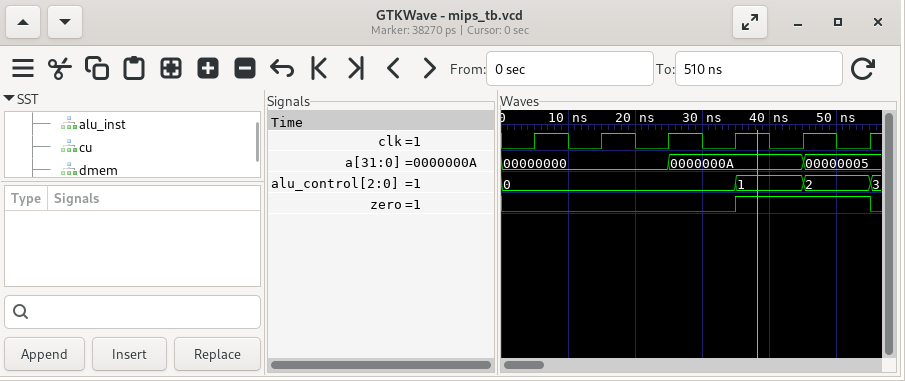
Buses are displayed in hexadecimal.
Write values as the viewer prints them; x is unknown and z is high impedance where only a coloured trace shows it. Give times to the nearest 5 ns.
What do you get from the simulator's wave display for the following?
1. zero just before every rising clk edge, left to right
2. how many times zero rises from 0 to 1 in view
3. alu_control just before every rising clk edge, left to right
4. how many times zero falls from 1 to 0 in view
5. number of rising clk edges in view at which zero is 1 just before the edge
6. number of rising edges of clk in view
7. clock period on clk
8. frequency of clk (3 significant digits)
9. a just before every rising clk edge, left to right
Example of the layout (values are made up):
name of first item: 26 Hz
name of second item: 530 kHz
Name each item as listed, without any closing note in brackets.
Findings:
zero just before every rising clk edge, left to right: 0 0 0 0 1 1
how many times zero rises from 0 to 1 in view: 1
alu_control just before every rising clk edge, left to right: 0, 0, 0, 0, 1, 2
how many times zero falls from 1 to 0 in view: 1
number of rising clk edges in view at which zero is 1 just before the edge: 2
number of rising edges of clk in view: 6
clock period on clk: 10 ns
frequency of clk: 100 MHz
a just before every rising clk edge, left to right: 00000000, 00000000, 00000000, 0000000A, 0000000A, 00000005
